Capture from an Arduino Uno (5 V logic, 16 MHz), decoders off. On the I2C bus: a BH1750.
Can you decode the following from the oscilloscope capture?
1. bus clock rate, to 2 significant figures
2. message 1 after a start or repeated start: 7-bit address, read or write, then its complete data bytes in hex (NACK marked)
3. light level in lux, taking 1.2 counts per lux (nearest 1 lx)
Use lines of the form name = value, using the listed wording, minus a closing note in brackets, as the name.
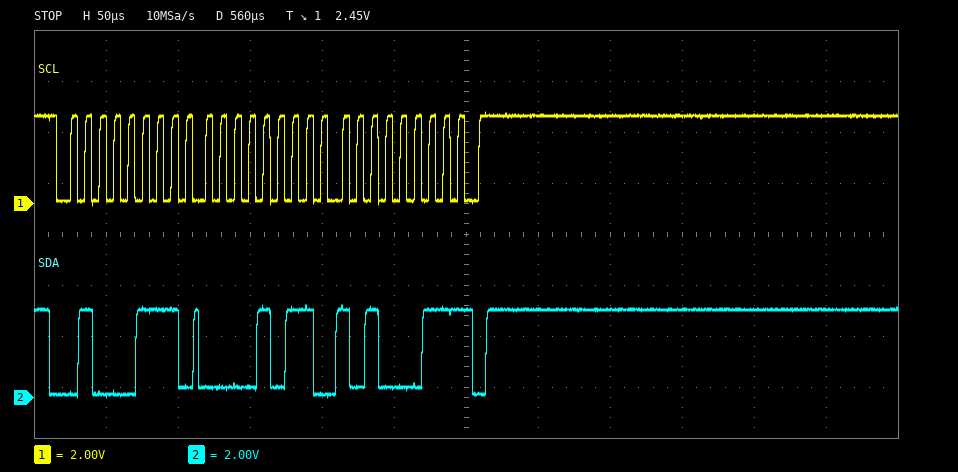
bus clock rate, to 2 significant figures = 100 kHz
message 1 after a start or repeated start: 7-bit address, read or write, then its complete data bytes in hex = 0x23 read: 0B A3 NACK
light level in lux, taking 1.2 counts per lux = 2482 lx
